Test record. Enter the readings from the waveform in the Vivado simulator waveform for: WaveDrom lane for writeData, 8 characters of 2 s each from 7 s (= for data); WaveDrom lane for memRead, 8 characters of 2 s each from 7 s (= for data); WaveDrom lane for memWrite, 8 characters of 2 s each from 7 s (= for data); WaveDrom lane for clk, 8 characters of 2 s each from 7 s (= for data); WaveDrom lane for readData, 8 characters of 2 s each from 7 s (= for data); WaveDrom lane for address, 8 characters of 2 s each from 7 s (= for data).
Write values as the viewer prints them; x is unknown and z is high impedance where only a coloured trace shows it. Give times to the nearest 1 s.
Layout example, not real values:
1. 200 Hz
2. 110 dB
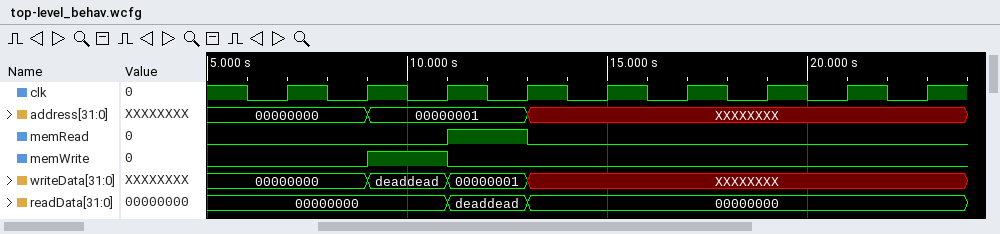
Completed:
1. {name: 'writeData', wave: '===x....', data: '00000000 deaddead 00000001'}
2. {name: 'memRead', wave: '0.10....'}
3. {name: 'memWrite', wave: '010.....'}
4. {name: 'clk', wave: 'p.......'}
5. {name: 'readData', wave: '=.==....', data: '00000000 deaddead 00000000'}
6. {name: 'address', wave: '==.x....', data: '00000000 00000001'}
